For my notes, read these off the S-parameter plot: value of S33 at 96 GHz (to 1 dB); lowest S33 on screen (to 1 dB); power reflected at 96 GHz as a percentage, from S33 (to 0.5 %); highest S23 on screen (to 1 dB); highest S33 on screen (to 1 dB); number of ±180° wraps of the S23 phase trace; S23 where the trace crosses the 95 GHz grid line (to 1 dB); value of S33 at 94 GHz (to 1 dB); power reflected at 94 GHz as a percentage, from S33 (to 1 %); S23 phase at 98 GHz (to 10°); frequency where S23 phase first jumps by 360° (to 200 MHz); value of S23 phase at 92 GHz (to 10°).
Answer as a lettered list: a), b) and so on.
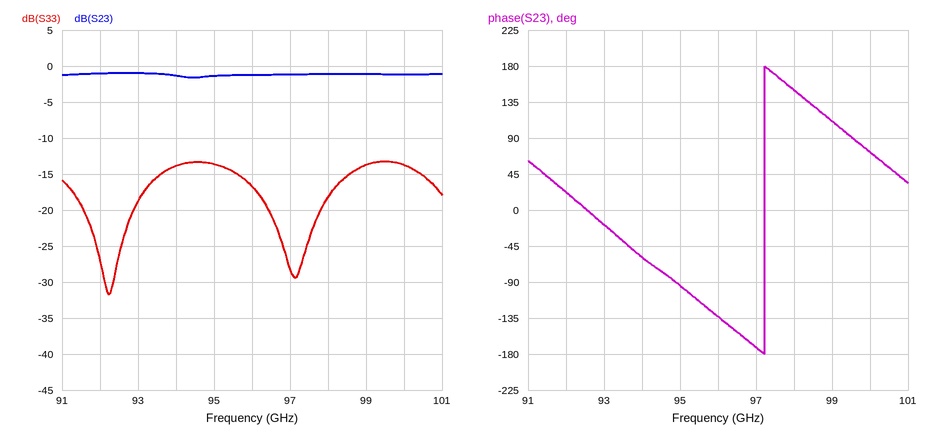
a) -17 dB
b) -32 dB
c) 2.0 %
d) -1 dB
e) -13 dB
f) 1
g) -1 dB
h) -14 dB
i) 4 %
j) 150°
k) 97.2 GHz
l) 20°
